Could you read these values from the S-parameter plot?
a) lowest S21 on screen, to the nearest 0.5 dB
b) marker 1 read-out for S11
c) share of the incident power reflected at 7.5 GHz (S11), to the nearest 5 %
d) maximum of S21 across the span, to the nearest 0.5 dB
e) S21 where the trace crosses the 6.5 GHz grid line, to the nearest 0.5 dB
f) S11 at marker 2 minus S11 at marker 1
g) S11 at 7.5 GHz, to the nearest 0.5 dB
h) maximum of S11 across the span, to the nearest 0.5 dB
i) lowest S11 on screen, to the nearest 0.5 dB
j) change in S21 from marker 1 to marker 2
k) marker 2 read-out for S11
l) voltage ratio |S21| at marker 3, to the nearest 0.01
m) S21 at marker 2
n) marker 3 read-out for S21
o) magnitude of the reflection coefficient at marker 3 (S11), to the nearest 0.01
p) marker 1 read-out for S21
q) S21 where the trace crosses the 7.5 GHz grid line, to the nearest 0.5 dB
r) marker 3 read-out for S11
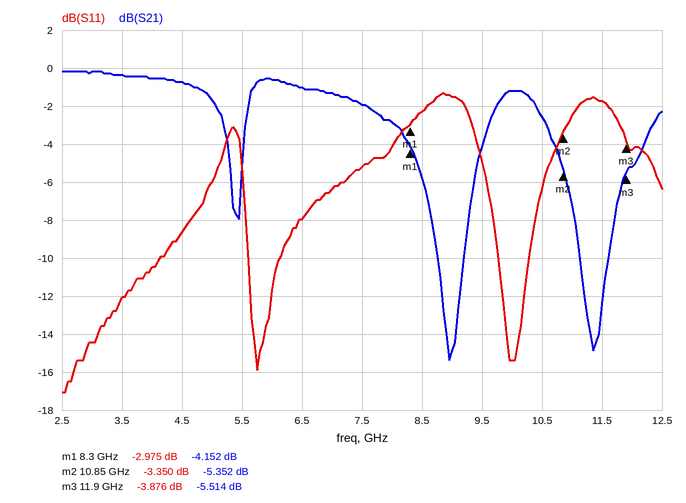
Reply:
-15.5 dB
-2.975 dB
30 %
0.0 dB
-1.0 dB
-0.375 dB
-5.0 dB
-1.5 dB
-17.0 dB
-1.200 dB
-3.350 dB
0.53
-5.352 dB
-5.514 dB
0.64
-4.152 dB
-2.0 dB
-3.876 dB
